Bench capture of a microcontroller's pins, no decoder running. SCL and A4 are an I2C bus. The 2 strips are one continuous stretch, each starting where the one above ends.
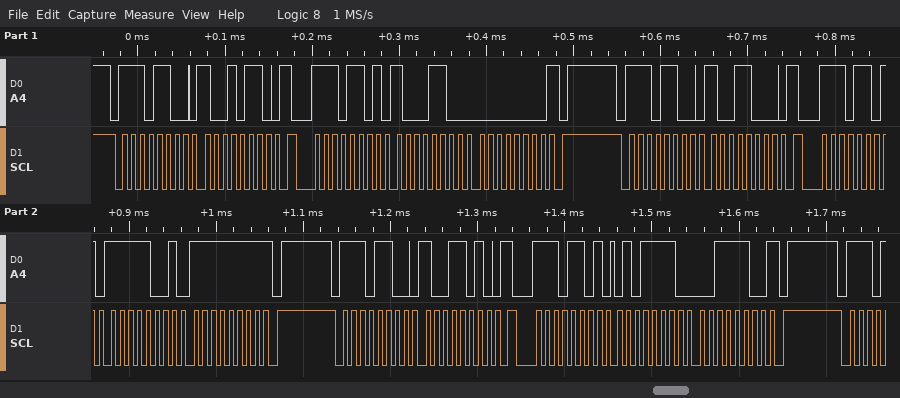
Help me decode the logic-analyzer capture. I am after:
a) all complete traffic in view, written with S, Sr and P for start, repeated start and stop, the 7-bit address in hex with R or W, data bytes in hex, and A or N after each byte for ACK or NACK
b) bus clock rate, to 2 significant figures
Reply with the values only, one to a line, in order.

S 76W A 96 A Sr 76R A 8C A 00 N P S 76W A 98 A Sr 76R A F9 A FF N P S 76W A 9A A Sr 76R A 5E A 3C N P
100 kHz
